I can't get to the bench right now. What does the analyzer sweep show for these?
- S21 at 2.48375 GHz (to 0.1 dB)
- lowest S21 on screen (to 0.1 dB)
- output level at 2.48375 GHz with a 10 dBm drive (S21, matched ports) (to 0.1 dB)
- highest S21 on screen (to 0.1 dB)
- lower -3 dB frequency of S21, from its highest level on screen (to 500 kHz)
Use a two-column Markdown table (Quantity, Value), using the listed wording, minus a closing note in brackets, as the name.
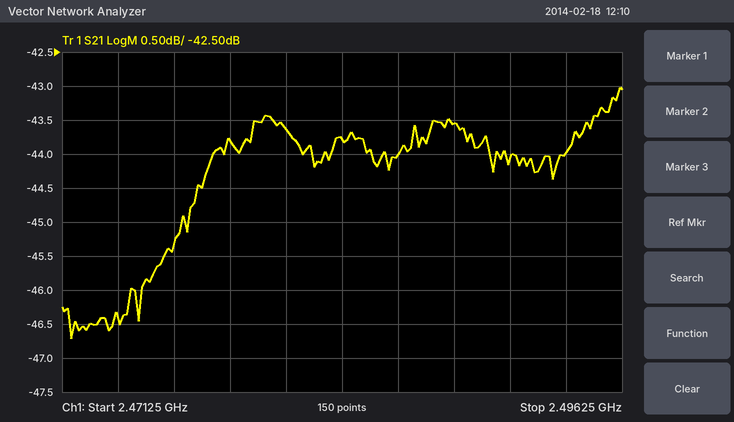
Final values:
| Quantity | Value |
|---|---|
| S21 at 2.48375 GHz | -43.8 dB |
| lowest S21 on screen | -46.7 dB |
| output level at 2.48375 GHz with a 10 dBm drive (S21, matched ports) | -33.8 dBm |
| highest S21 on screen | -43.0 dB |
| lower -3 dB frequency of S21, from its highest level on screen | 2.4750 GHz |
